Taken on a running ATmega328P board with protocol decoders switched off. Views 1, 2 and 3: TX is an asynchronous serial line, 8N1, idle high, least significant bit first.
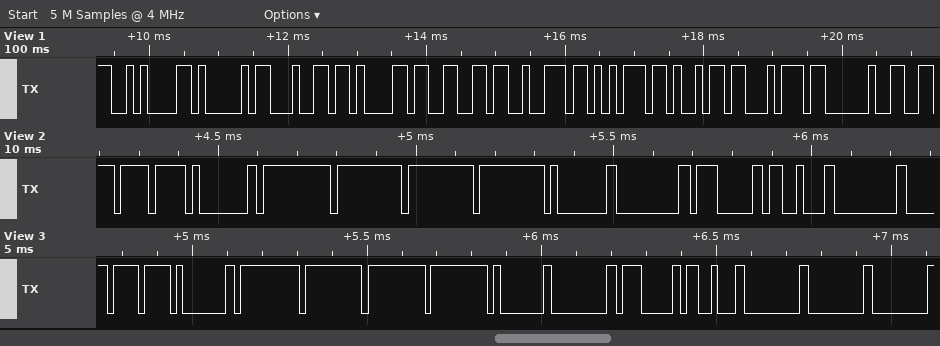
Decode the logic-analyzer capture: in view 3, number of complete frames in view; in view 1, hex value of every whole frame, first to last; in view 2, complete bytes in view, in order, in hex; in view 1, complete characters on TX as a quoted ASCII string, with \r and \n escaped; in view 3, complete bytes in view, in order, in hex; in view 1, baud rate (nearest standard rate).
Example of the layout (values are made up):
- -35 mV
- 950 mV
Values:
- 13
- 0x0A 0x41 0x64 0x61 0x66 0x72 0x75 0x69 0x74 0x20
- EF 01 FF FF FF FF 01 00 07 13 00
- "\nAdafruit "
- 0xEF 0x01 0xFF 0xFF 0xFF 0xFF 0x01 0x00 0x07 0x13 0x00 0x00 0x00
- 9600 baud
